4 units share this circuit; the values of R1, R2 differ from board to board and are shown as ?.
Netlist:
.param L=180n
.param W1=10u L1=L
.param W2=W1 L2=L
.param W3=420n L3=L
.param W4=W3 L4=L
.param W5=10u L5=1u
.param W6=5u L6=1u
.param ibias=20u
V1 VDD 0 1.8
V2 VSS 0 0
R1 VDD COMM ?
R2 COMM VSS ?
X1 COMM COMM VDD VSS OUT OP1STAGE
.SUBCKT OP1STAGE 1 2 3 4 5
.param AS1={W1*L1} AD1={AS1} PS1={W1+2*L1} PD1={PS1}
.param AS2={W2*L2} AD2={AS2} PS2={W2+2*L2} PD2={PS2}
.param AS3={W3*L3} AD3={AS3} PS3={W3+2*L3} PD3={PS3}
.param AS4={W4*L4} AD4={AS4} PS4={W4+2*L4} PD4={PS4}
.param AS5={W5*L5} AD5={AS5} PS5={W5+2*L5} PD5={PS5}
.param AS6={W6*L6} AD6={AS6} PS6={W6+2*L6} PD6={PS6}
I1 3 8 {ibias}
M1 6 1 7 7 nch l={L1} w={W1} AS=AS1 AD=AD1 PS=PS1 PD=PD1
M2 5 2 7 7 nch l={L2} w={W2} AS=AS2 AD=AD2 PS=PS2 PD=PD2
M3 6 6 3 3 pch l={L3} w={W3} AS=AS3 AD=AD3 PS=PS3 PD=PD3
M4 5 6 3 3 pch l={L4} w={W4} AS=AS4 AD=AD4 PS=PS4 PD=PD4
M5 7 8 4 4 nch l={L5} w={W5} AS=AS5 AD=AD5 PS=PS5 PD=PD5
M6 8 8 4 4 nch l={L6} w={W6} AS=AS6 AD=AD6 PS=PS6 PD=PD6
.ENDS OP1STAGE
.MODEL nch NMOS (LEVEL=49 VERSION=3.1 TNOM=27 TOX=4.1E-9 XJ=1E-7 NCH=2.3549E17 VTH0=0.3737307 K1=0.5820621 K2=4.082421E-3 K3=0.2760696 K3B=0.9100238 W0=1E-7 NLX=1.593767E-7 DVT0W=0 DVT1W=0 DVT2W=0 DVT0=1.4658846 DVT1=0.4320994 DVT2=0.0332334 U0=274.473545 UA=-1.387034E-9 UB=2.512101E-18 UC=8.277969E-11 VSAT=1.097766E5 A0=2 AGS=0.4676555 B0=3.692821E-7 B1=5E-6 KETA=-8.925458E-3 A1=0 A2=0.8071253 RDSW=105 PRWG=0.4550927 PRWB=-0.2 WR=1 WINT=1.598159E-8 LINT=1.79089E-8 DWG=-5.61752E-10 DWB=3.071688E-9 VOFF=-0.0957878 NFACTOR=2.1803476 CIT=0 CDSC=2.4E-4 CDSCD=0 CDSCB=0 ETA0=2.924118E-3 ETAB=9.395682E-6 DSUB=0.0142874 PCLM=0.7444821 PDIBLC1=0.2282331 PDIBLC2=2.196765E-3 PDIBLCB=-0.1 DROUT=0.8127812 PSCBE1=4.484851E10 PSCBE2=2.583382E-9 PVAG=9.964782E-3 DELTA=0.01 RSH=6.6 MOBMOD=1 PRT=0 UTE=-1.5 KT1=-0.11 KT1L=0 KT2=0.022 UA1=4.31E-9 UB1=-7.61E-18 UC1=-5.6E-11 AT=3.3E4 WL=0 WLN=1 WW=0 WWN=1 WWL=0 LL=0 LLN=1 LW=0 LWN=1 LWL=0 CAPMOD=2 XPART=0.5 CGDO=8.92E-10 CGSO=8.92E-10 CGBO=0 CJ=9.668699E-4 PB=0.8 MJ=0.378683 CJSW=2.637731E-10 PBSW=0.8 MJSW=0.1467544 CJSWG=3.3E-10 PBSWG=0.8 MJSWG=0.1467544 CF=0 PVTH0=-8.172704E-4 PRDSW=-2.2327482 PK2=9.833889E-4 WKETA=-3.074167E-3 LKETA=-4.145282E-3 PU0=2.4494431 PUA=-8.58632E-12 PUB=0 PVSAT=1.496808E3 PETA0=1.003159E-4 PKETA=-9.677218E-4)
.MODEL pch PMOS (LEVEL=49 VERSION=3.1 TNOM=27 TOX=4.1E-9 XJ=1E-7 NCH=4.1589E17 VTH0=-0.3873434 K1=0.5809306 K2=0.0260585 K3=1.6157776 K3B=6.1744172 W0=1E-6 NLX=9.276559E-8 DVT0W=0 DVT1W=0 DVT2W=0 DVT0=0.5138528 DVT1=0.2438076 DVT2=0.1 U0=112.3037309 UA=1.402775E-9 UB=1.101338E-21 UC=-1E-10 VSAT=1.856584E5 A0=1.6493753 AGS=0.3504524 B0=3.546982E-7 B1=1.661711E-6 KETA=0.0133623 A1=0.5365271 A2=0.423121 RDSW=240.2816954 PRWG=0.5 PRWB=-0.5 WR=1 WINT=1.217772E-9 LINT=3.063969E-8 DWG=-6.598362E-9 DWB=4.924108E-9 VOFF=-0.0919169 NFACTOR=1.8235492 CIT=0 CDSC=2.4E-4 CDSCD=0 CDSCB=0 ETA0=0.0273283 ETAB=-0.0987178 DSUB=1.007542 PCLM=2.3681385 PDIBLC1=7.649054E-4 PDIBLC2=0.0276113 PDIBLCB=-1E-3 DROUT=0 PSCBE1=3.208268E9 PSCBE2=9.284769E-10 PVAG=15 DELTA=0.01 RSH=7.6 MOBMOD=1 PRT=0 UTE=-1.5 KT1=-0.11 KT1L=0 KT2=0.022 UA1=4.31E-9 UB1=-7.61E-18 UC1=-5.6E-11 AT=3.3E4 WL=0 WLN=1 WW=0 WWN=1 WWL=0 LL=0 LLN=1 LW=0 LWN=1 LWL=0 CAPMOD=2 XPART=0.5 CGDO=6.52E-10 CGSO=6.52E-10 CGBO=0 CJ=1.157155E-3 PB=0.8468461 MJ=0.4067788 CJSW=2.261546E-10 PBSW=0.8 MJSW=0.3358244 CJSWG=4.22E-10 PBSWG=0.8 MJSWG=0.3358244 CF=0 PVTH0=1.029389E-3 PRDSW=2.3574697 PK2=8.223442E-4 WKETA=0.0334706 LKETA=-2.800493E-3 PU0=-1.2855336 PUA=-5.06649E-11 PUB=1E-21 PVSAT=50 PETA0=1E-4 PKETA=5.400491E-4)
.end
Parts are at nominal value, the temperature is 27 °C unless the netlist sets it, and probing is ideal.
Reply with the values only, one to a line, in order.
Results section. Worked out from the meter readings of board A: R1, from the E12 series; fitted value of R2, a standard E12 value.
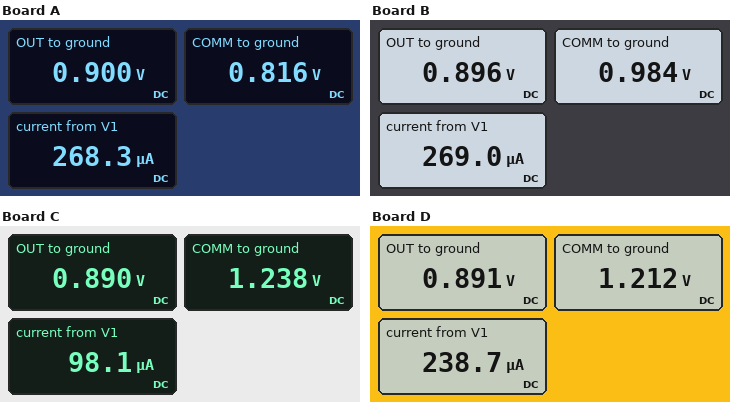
4.7 kΩ
3.9 kΩ
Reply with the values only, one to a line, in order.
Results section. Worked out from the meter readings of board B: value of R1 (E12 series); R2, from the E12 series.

3.9 kΩ
4.7 kΩ
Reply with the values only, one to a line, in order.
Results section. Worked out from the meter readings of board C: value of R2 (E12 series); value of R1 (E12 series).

33 kΩ
15 kΩ
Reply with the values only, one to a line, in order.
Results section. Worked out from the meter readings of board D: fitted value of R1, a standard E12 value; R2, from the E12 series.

3.3 kΩ
6.8 kΩ
